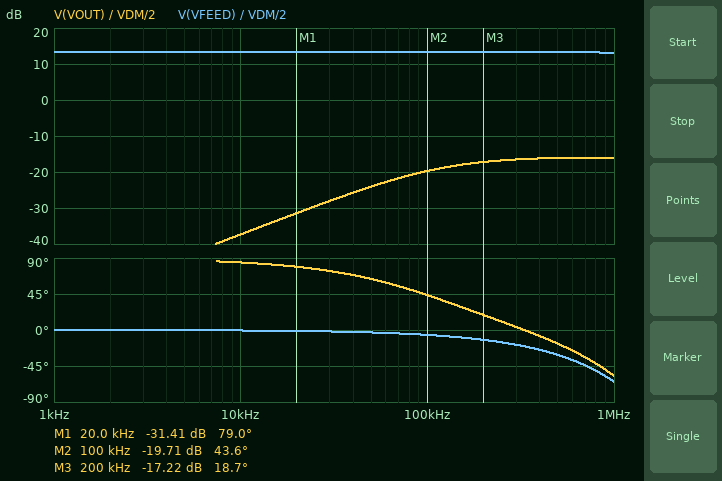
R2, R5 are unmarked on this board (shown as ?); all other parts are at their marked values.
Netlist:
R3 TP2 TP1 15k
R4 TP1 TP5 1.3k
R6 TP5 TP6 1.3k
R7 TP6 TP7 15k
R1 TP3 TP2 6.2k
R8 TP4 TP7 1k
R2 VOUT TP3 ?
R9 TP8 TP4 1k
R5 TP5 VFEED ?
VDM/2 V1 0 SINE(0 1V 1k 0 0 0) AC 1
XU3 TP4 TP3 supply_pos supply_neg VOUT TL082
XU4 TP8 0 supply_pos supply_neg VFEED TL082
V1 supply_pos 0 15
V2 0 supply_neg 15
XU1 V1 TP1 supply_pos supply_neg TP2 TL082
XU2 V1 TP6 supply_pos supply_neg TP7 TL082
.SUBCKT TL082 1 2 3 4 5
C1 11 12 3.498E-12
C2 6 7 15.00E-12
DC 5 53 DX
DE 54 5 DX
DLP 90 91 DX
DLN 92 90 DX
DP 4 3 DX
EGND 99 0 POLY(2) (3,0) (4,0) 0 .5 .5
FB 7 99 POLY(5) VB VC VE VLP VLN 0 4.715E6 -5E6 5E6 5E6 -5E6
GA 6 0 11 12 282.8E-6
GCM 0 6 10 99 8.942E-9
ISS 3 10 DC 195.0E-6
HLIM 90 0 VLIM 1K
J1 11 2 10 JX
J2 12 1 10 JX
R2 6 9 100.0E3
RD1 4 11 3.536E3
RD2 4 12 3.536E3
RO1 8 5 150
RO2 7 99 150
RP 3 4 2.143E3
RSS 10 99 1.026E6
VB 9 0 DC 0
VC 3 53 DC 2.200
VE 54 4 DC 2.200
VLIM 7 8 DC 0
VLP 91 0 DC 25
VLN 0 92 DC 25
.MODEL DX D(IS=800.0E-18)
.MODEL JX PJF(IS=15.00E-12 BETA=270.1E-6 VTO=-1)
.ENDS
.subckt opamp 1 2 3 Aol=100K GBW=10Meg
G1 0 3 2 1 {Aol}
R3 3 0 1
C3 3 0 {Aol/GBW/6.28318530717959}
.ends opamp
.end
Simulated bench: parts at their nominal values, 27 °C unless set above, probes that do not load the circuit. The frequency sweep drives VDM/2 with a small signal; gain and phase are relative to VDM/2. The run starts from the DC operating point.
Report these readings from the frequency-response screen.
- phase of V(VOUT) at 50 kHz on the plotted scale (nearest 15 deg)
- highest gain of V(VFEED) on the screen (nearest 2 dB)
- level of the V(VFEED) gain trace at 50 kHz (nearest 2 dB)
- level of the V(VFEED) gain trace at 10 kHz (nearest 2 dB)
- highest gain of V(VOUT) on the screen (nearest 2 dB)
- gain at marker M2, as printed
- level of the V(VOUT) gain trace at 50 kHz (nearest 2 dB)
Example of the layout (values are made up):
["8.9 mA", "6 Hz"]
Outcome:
["60 deg", "14 dB", "14 dB", "14 dB", "-16 dB", "-19.71 dB", "-24 dB"]
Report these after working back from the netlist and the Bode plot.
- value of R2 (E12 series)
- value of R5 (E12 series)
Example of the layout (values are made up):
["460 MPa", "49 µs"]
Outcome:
["180 kΩ", "27 kΩ"]
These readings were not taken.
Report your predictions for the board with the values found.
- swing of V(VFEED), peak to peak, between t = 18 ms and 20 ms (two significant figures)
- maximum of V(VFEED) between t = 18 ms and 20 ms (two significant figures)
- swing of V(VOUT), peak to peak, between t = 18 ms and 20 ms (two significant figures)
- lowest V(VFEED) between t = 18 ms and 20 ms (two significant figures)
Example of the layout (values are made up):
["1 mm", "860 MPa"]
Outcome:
["9.4 V", "4.7 V", "2.7 mV", "-4.7 V"]
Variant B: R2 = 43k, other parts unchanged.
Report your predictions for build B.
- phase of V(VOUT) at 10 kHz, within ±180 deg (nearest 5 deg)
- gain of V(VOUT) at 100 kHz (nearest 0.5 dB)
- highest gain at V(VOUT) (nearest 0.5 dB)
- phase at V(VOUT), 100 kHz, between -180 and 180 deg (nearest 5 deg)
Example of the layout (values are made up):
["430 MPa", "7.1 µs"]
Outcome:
["90 deg", "-17.5 dB", "-5.0 dB", "70 deg"]
